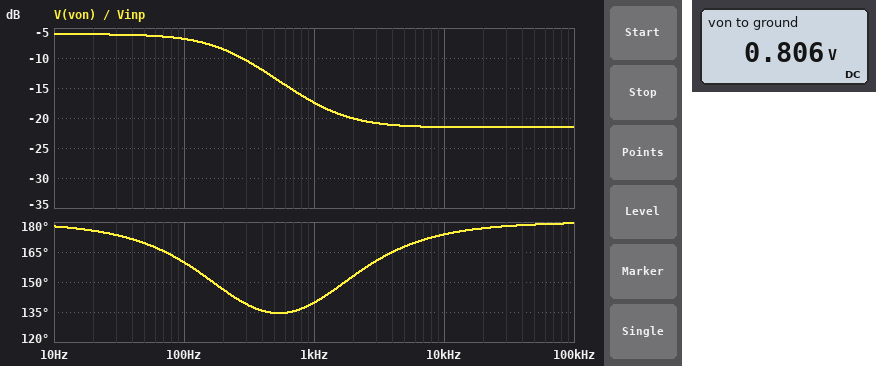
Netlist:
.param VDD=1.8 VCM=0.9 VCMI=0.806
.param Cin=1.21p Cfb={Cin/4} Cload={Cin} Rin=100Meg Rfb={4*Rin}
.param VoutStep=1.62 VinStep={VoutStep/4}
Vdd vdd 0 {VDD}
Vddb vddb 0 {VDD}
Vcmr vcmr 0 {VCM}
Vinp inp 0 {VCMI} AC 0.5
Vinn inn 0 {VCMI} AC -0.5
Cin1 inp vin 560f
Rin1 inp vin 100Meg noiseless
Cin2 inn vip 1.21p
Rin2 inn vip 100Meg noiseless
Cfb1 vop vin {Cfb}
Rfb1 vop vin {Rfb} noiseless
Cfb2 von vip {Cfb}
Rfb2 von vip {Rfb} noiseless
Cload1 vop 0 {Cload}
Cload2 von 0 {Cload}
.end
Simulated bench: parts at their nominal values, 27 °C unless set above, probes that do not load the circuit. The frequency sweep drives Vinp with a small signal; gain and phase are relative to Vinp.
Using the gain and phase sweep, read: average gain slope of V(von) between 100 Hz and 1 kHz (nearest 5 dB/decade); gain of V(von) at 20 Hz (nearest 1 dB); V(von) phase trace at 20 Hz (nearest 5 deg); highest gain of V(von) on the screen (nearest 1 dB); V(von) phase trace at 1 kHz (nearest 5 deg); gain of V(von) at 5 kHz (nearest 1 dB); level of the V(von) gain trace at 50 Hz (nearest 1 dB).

-10 dB/decade
-6 dB
175 deg
-6 dB
140 deg
-21 dB
-6 dB
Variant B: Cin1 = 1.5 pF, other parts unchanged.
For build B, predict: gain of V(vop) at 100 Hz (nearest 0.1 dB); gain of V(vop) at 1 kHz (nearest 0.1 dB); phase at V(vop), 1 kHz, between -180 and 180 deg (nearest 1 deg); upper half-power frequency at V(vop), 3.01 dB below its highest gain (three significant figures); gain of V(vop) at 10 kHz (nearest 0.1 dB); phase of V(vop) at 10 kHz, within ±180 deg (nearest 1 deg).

-0.8 dB
-11.3 dB
-39 deg
224 Hz
-15.2 dB
-6 deg
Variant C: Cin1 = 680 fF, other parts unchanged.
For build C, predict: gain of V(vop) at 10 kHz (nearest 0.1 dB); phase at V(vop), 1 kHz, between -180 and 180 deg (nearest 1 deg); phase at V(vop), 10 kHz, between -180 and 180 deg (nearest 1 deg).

-16.5 dB
-43 deg
-8 deg
